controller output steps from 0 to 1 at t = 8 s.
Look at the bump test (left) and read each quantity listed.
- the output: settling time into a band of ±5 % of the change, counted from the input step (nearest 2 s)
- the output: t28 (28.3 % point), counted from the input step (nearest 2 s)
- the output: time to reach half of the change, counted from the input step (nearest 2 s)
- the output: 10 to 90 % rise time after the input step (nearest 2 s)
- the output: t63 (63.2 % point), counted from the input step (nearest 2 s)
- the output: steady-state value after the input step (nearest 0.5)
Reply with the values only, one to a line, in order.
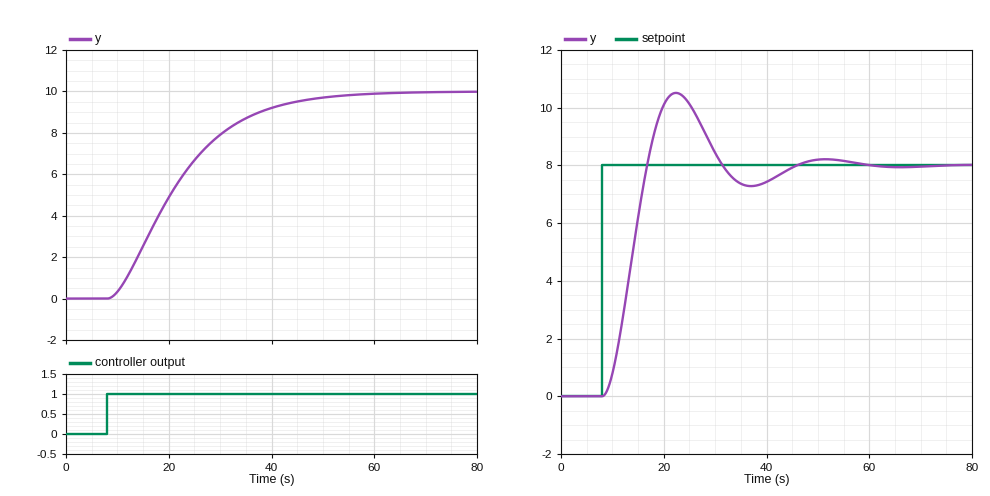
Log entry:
36 s
8 s
12 s
26 s
16 s
10.0
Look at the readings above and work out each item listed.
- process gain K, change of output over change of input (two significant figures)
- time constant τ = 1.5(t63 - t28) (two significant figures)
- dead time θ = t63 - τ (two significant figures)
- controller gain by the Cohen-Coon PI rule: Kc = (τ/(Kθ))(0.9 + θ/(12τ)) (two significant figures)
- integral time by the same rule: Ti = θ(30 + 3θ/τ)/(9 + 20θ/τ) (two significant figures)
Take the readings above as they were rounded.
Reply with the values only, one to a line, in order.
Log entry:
10
12 s
4.0 s
0.28
7.9 s
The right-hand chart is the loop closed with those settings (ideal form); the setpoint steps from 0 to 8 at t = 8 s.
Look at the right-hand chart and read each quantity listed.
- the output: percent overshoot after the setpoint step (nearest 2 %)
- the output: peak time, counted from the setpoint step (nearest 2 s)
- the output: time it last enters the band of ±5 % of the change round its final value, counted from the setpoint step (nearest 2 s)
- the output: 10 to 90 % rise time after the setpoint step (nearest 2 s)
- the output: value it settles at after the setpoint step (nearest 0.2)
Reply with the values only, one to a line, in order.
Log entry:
32 %
14 s
34 s
6 s
8.0
